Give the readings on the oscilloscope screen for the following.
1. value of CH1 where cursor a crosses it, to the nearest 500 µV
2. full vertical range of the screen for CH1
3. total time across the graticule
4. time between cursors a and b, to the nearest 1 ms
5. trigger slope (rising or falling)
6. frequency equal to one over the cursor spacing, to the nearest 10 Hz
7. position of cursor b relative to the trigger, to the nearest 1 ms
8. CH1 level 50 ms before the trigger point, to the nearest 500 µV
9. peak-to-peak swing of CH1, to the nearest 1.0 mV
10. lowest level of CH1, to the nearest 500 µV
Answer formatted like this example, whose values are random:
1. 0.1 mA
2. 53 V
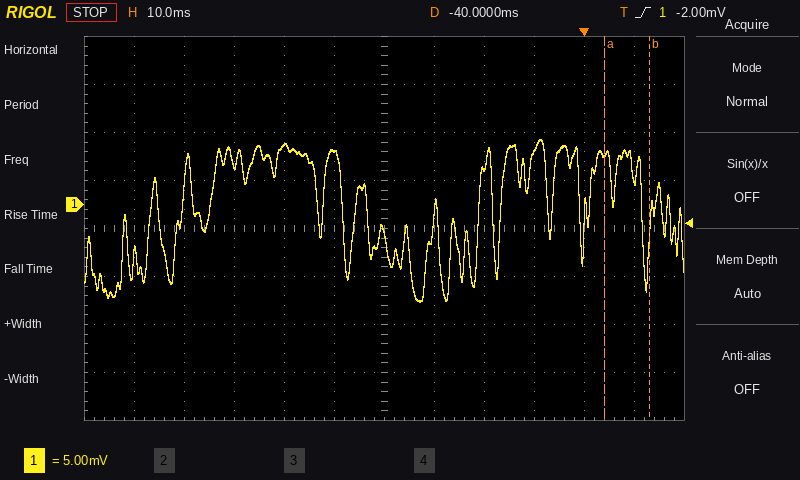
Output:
1. 5.5 mV
2. 40 mV
3. 120 ms
4. 9 ms
5. rising
6. 110 Hz
7. +13 ms
8. 5.5 mV
9. 17.0 mV
10. -10.0 mV
